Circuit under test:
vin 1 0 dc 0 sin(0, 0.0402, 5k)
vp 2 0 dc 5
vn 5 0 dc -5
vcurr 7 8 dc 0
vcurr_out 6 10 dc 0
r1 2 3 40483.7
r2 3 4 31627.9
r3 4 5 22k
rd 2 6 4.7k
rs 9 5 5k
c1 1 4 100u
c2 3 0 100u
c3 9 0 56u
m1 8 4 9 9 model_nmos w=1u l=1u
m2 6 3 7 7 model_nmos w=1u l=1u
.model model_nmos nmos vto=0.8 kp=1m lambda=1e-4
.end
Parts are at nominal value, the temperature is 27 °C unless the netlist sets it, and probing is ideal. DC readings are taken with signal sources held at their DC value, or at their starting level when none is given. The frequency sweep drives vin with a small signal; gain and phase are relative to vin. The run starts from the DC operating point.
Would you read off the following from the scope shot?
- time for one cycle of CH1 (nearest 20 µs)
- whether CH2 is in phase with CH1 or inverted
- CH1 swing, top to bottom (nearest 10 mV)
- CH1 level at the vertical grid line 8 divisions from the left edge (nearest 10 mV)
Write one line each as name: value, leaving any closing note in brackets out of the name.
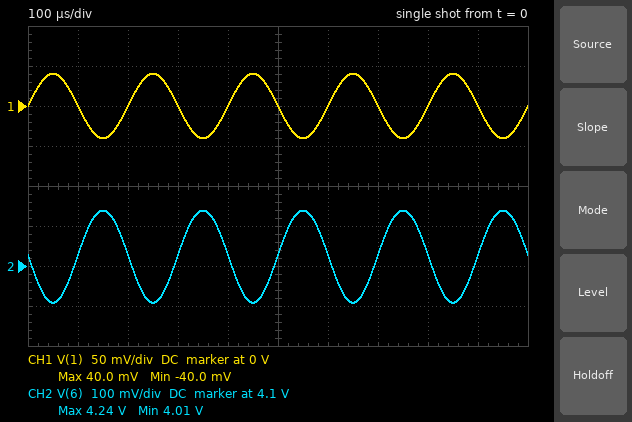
time for one cycle of CH1: 200 µs
whether CH2 is in phase with CH1 or inverted: inverted
CH1 swing, top to bottom: 80 mV
CH1 level at the vertical grid line 8 divisions from the left edge: 0 V
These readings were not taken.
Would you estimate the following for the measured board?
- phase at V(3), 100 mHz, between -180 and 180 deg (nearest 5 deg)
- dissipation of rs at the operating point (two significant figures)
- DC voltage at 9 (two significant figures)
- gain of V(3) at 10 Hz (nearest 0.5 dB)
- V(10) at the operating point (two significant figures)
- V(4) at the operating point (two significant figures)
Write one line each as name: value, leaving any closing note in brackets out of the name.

phase at V(3), 100 mHz, between -180 and 180 deg: -5 deg
dissipation of rs at the operating point: 170 µW
DC voltage at 9: -4.1 V
gain of V(3) at 10 Hz: -46.0 dB
V(10) at the operating point: 4.1 V
V(4) at the operating point: -2.7 V
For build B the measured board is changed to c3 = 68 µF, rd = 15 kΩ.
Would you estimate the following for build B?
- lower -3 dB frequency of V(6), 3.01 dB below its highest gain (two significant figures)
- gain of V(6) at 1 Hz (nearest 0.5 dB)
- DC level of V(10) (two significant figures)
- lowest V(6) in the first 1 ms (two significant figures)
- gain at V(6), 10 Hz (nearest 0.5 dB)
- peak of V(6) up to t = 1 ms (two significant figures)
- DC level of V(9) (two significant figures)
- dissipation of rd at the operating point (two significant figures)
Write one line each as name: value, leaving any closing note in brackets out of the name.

lower -3 dB frequency of V(6), 3.01 dB below its highest gain: 1.8 Hz
gain of V(6) at 1 Hz: 13.5 dB
DC level of V(10): 2.2 V
lowest V(6) in the first 1 ms: 1.8 V
gain at V(6), 10 Hz: 19.0 dB
peak of V(6) up to t = 1 ms: 2.6 V
DC level of V(9): -4.1 V
dissipation of rd at the operating point: 520 µW
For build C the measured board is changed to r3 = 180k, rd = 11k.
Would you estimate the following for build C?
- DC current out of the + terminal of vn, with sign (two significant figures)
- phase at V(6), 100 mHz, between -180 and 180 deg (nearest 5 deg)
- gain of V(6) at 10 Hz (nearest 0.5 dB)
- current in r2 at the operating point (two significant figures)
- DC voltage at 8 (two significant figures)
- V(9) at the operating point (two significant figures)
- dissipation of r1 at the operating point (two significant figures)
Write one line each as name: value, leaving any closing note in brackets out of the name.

DC current out of the + terminal of vn, with sign: -640 µA
phase at V(6), 100 mHz, between -180 and 180 deg: -160 deg
gain of V(6) at 10 Hz: -24.5 dB
current in r2 at the operating point: 40 µA
DC voltage at 8: -1.8 V
V(9) at the operating point: -2.0 V
dissipation of r1 at the operating point: 64 µW
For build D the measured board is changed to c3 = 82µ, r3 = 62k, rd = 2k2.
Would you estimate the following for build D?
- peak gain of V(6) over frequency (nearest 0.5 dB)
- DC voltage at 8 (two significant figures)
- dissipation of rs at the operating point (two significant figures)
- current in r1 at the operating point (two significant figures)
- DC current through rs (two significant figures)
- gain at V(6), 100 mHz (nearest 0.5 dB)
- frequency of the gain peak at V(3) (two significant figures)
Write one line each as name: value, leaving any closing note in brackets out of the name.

peak gain of V(6) over frequency: 7.5 dB
DC voltage at 8: 130 mV
dissipation of rs at the operating point: 1.5 mW
current in r1 at the operating point: 75 µA
DC current through rs: 550 µA
gain at V(6), 100 mHz: -10.5 dB
frequency of the gain peak at V(3): 65 mHz
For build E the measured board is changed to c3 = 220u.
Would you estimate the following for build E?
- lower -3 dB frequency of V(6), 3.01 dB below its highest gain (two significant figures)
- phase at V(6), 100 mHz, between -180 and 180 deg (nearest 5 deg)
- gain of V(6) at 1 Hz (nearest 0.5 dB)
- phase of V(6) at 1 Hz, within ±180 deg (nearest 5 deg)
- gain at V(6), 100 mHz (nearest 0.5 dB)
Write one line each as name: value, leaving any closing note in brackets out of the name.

lower -3 dB frequency of V(6), 3.01 dB below its highest gain: 580 mHz
phase at V(6), 100 mHz, between -180 and 180 deg: -110 deg
gain of V(6) at 1 Hz: 8.0 dB
phase of V(6) at 1 Hz, within ±180 deg: -150 deg
gain at V(6), 100 mHz: -5.5 dB
